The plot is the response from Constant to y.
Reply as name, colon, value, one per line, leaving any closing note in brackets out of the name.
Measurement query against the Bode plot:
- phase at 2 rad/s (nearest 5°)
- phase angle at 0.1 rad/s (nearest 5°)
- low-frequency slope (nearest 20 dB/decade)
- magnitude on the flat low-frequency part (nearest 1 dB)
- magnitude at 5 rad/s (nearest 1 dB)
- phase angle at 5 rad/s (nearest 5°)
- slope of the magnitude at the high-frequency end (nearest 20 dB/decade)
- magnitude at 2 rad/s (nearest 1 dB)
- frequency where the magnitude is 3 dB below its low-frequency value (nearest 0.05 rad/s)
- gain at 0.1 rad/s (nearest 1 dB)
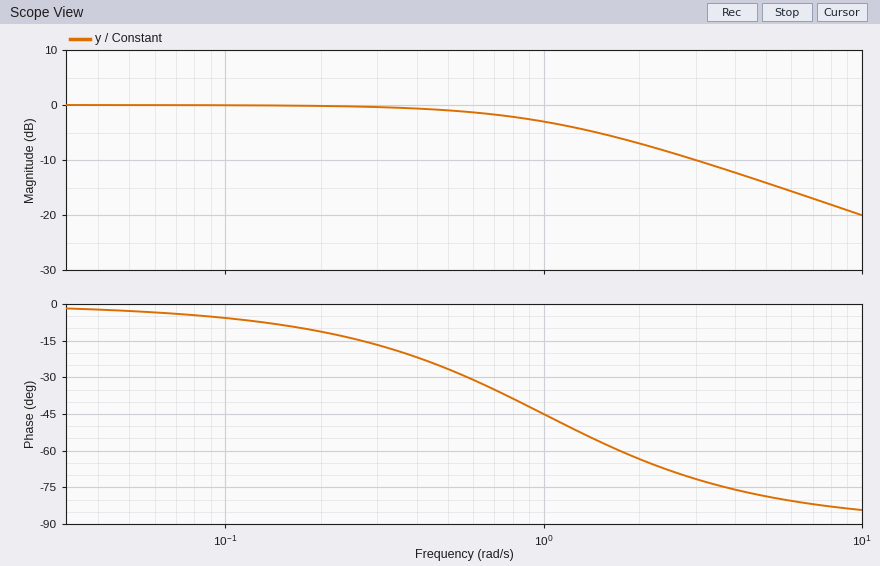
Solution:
phase at 2 rad/s: -65°
phase angle at 0.1 rad/s: -5°
low-frequency slope: 0 dB/decade
magnitude on the flat low-frequency part: 0 dB
magnitude at 5 rad/s: -14 dB
phase angle at 5 rad/s: -80°
slope of the magnitude at the high-frequency end: -20 dB/decade
magnitude at 2 rad/s: -7 dB
frequency where the magnitude is 3 dB below its low-frequency value: 1.00 rad/s
gain at 0.1 rad/s: 0 dB
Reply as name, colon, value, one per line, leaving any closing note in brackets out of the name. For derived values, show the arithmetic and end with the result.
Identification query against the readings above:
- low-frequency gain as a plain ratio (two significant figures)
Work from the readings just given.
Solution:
low-frequency gain as a plain ratio: 10^(0 / 20) = 1.0
